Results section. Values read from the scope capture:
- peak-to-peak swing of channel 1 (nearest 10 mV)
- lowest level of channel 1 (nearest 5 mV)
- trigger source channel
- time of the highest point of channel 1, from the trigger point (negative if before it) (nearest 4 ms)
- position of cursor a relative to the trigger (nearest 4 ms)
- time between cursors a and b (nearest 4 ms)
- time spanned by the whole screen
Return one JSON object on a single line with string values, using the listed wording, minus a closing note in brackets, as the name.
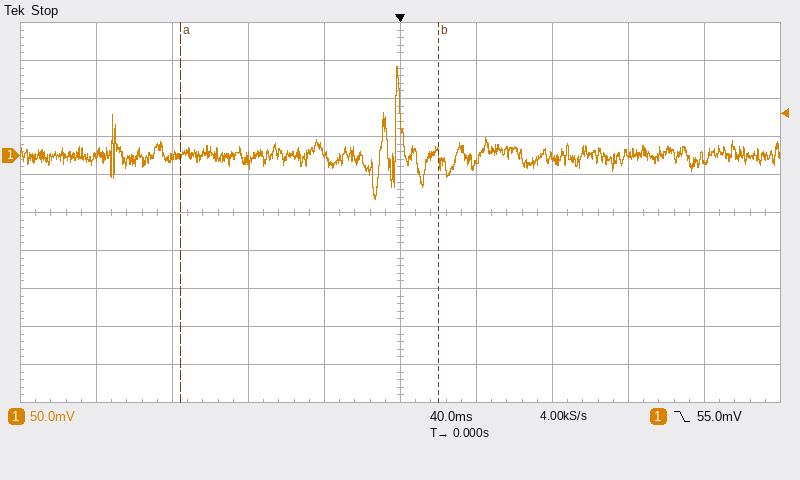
{"peak-to-peak swing of channel 1": "180 mV", "lowest level of channel 1": "-60 mV", "trigger source channel": "channel 1", "time of the highest point of channel 1, from the trigger point (negative if before it)": "0 ms", "position of cursor a relative to the trigger": "-116 ms", "time between cursors a and b": "136 ms", "time spanned by the whole screen": "400 ms"}
